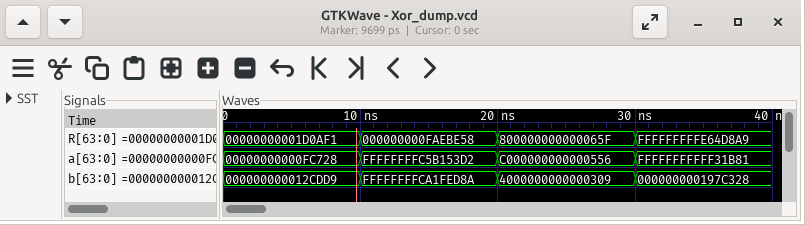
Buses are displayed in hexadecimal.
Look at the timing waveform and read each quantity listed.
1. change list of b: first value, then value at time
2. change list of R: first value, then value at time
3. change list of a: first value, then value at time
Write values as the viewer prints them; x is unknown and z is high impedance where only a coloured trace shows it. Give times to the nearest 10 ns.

000000000012CDD9, FFFFFFFFCA1FED8A at 10 ns, 4000000000000309 at 20 ns, 000000000197C328 at 30 ns
00000000001D0AF1, 000000000FAEBE58 at 10 ns, 800000000000065F at 20 ns, FFFFFFFFFE64D8A9 at 30 ns
00000000000FC728, FFFFFFFFC5B153D2 at 10 ns, C000000000000556 at 20 ns, FFFFFFFFFFF31B81 at 30 ns
